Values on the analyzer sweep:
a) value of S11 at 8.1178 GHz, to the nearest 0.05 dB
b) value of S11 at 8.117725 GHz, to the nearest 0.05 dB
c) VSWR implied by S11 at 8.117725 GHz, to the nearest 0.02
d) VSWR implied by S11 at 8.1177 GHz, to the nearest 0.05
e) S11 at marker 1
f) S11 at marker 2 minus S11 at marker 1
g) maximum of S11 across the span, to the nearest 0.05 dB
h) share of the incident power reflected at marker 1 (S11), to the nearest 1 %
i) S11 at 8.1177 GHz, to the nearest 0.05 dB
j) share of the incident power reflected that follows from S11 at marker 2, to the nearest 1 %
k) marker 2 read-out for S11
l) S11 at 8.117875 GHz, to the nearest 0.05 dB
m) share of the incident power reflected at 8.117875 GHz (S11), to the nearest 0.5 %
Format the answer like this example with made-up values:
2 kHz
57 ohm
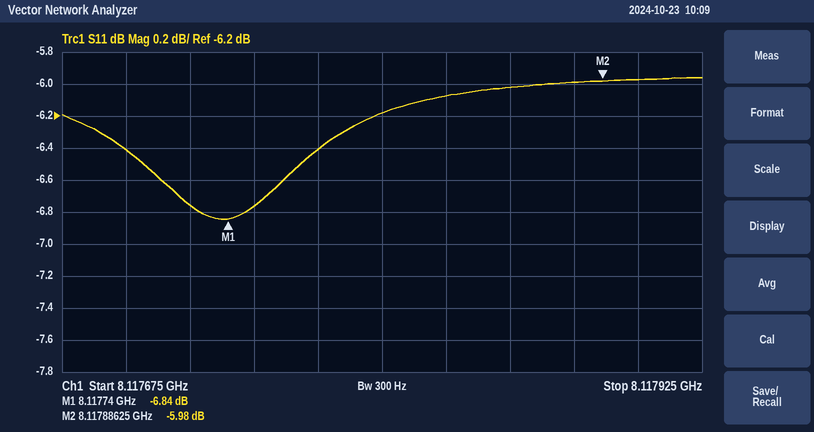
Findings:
-6.20 dB
-6.75 dB
2.70
2.85
-6.84 dB
0.86 dB
-5.95 dB
21 %
-6.40 dB
25 %
-5.98 dB
-6.00 dB
25.0 %
